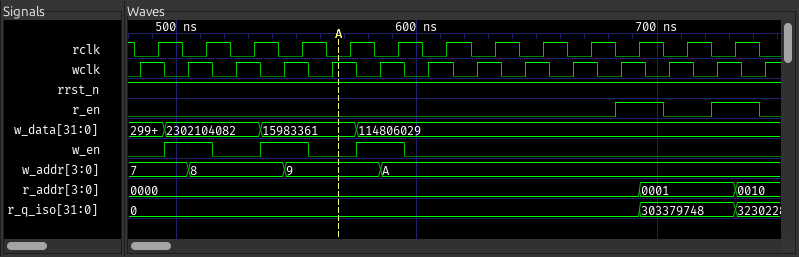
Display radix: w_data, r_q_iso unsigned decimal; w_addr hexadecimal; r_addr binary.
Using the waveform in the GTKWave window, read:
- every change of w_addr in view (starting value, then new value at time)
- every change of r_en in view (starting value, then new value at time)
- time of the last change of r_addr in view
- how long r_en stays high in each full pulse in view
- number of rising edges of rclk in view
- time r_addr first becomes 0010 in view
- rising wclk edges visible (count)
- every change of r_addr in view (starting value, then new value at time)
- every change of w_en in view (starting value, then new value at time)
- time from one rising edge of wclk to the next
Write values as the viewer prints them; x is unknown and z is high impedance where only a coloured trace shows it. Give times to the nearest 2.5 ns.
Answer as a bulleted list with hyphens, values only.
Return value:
- 7, 8 at 505 ns, 9 at 545 ns, A at 585 ns
- 0, 1 at 682.5 ns, 0 at 702.5 ns, 1 at 722.5 ns, 0 at 742.5 ns
- 732.5 ns
- 20 ns, 20 ns
- 13
- 732.5 ns
- 14
- 0000, 0001 at 692.5 ns, 0010 at 732.5 ns
- 0, 1 at 495 ns, 0 at 515 ns, 1 at 535 ns, 0 at 555 ns, 1 at 575 ns, 0 at 595 ns
- 20 ns
